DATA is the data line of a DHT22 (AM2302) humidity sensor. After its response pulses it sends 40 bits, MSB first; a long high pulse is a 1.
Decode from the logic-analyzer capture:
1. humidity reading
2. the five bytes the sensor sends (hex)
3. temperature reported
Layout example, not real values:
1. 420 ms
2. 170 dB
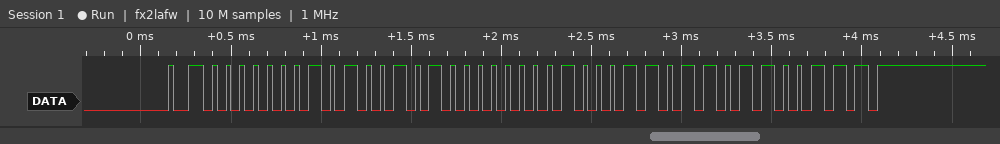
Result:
1. 33.0 %
2. 01 4A 01 1B 67
3. 28.3 °C
